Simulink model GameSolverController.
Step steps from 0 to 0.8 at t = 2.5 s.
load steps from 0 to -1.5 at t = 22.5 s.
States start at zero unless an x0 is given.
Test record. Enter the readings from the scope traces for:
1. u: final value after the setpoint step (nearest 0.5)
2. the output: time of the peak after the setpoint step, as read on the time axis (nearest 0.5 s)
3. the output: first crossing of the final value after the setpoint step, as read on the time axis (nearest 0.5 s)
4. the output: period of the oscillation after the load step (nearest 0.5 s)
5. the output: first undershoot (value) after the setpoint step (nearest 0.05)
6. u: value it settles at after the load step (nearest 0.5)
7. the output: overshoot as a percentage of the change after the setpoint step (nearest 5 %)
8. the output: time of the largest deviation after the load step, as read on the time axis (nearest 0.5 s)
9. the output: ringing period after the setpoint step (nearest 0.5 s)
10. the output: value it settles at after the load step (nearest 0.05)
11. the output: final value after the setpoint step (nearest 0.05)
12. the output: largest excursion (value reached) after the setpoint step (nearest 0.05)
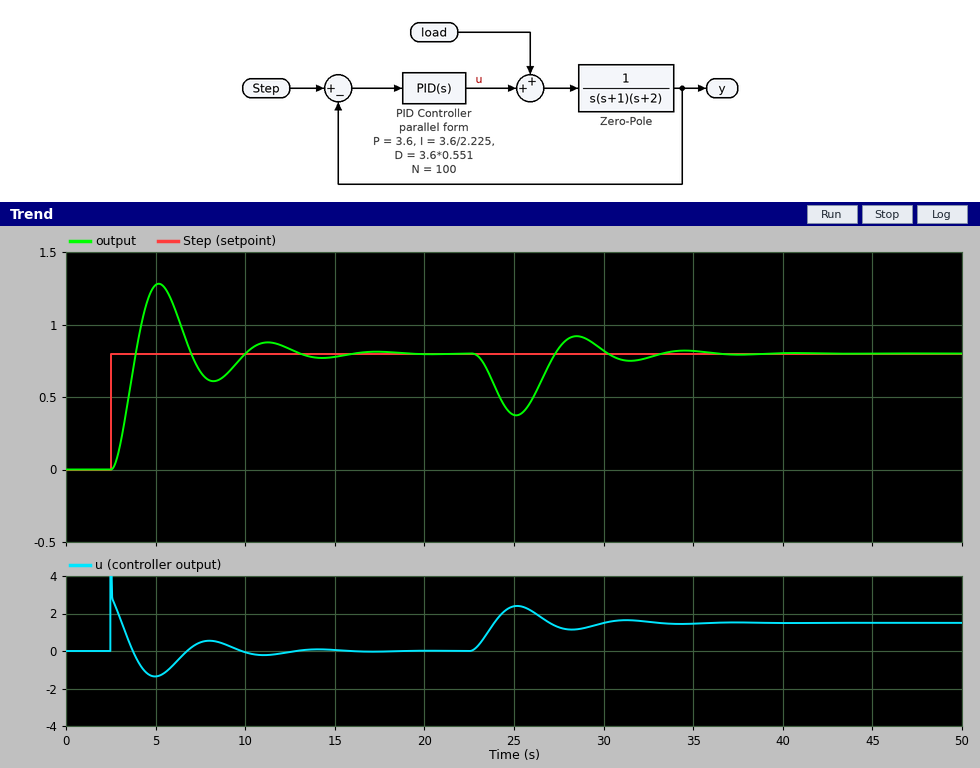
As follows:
0.0
5.0 s
4.0 s
6.5 s
0.60
1.5
60 %
25.0 s
6.0 s
0.80
0.80
1.30
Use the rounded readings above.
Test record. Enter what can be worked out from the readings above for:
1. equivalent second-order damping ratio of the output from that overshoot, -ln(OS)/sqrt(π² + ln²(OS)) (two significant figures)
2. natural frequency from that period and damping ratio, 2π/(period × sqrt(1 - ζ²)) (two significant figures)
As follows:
0.16
1.1 rad/s
